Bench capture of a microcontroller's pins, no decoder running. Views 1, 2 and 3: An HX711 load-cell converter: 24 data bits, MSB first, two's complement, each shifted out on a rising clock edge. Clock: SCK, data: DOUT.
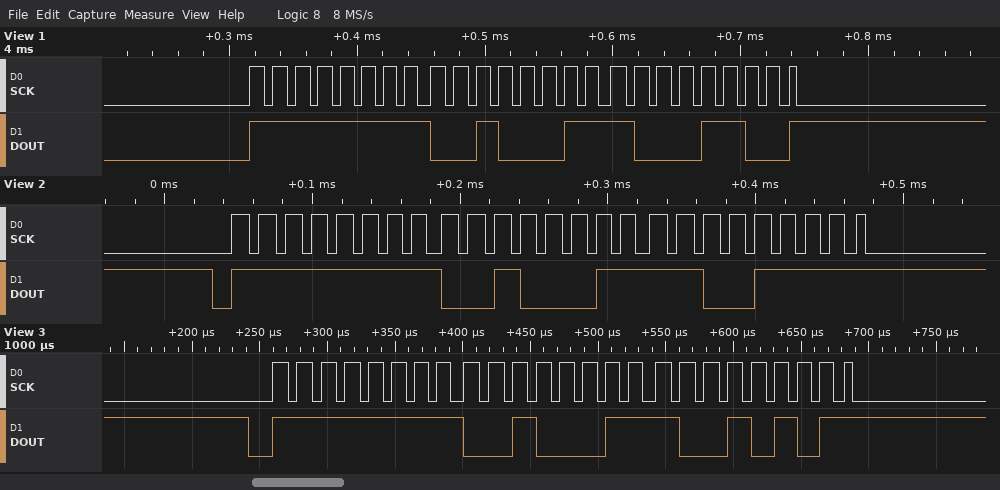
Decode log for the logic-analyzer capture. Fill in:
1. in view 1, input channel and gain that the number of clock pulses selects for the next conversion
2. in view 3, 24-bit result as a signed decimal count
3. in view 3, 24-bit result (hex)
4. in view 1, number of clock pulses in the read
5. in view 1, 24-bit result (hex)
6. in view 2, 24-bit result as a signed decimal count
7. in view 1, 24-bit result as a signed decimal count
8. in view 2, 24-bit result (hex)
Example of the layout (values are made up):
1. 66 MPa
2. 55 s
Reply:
1. channel A, gain 128
2. -56427
3. 0xFF2395
4. 25
5. 0xFF238C
6. -56369
7. -56436
8. 0xFF23CF
